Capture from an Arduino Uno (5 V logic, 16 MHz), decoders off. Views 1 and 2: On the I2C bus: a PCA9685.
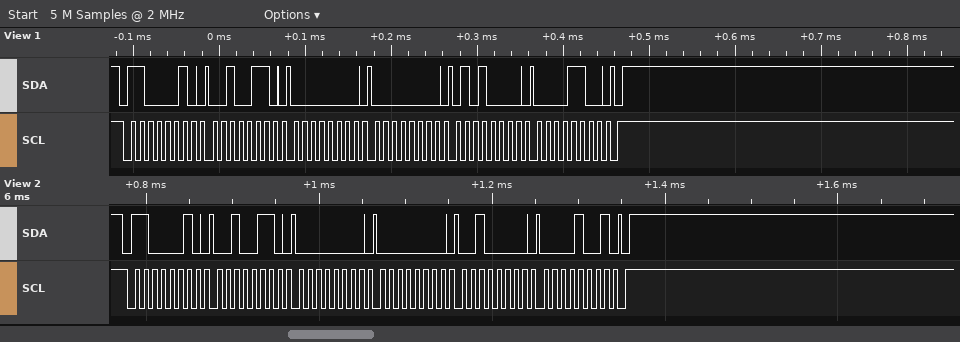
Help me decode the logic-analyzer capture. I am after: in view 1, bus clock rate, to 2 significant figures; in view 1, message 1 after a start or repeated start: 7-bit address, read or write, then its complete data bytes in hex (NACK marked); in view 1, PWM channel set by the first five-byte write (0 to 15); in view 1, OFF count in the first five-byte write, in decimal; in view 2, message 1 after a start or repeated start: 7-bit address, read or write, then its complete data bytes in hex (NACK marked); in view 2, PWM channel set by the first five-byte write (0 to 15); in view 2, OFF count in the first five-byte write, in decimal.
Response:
100 kHz
0x61 write: 26 00 00 50 0C
8
3152
0x61 write: 26 00 00 20 09
8
2336
